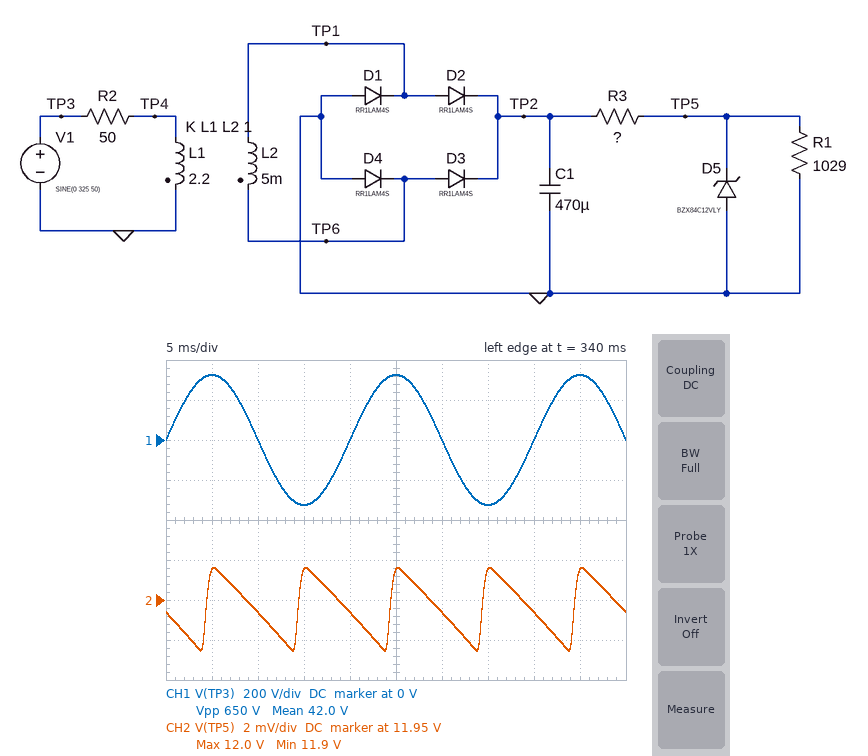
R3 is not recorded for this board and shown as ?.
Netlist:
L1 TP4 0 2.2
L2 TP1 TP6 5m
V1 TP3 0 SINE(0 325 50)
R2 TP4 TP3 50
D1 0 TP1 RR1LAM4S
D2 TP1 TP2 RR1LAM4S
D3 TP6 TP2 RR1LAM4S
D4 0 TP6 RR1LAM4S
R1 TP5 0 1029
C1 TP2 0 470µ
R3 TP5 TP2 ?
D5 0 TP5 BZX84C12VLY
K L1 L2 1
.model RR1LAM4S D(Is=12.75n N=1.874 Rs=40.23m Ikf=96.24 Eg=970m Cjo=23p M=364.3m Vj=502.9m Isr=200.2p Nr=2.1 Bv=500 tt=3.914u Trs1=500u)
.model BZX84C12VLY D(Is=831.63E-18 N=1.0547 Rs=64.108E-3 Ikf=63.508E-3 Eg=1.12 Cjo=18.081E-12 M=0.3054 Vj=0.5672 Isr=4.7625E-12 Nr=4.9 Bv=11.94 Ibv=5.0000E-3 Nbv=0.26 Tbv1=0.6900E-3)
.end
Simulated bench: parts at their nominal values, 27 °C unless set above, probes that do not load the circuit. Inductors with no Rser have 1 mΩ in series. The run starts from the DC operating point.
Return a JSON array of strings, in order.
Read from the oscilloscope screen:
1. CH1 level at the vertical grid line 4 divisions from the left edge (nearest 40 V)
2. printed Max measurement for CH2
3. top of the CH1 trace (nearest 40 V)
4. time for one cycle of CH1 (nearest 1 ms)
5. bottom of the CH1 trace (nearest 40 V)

["0 V", "12.0 V", "320 V", "20 ms", "-320 V"]
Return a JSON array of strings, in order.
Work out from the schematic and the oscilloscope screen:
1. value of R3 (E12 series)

["56 Ω"]
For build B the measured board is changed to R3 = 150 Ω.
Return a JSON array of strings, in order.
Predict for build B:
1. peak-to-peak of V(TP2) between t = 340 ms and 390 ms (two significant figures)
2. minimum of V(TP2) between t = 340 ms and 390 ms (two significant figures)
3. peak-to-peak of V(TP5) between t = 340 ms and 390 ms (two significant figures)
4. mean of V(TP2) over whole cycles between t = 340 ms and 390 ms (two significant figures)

["230 mV", "14 V", "14 mV", "14 V"]
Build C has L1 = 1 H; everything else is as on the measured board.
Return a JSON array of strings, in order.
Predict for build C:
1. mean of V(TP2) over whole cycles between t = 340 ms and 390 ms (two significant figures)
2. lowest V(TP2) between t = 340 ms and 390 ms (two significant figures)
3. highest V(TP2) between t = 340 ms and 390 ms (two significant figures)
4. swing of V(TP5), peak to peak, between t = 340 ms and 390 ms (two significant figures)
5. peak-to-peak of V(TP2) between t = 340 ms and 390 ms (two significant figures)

["20 V", "19 V", "21 V", "4.9 mV", "2.4 V"]
